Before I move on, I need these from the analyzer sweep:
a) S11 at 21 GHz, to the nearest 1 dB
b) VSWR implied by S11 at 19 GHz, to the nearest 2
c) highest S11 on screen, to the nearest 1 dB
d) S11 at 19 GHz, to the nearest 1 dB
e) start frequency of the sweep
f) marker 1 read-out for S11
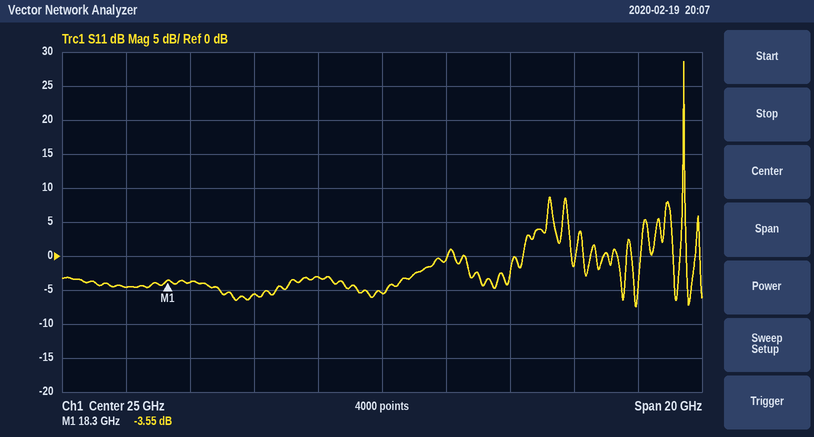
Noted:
-6 dB
4
29 dB
-4 dB
15 GHz
-3.55 dB
